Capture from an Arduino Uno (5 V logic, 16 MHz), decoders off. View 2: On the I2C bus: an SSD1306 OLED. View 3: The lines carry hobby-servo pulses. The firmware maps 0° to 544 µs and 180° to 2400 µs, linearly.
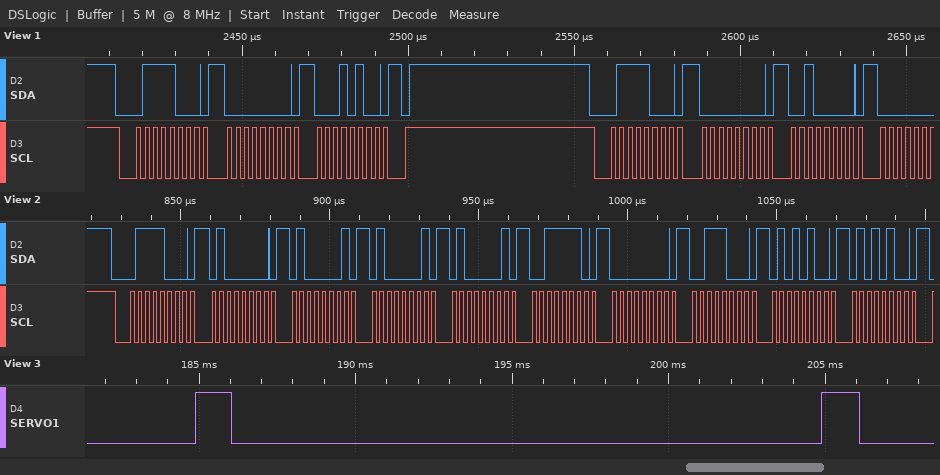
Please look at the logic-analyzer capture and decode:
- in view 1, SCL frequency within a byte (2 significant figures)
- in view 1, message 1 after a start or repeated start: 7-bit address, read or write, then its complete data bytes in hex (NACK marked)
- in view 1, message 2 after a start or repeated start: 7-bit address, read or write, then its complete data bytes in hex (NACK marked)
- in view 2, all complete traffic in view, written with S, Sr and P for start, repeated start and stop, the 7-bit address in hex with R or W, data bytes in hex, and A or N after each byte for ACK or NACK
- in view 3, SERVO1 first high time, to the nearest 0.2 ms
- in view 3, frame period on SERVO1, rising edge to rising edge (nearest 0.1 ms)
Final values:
400 kHz
0x3C write: 00 14
0x3C write: 00 20
S 3CW A 40 A 41 A 41 A 41 A 3E A 00 A 38 A 54 A 54 A
1.2 ms
20.0 ms
